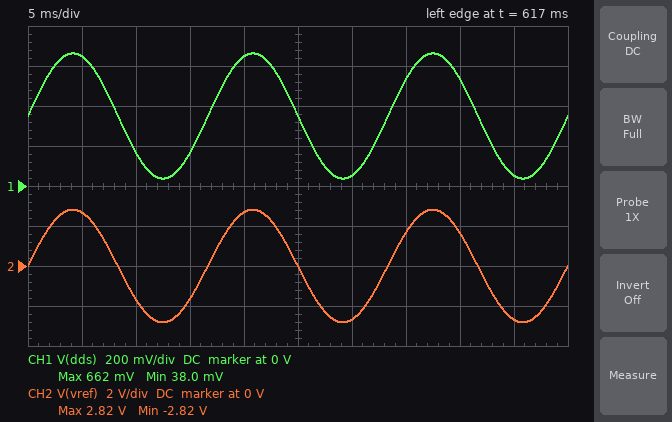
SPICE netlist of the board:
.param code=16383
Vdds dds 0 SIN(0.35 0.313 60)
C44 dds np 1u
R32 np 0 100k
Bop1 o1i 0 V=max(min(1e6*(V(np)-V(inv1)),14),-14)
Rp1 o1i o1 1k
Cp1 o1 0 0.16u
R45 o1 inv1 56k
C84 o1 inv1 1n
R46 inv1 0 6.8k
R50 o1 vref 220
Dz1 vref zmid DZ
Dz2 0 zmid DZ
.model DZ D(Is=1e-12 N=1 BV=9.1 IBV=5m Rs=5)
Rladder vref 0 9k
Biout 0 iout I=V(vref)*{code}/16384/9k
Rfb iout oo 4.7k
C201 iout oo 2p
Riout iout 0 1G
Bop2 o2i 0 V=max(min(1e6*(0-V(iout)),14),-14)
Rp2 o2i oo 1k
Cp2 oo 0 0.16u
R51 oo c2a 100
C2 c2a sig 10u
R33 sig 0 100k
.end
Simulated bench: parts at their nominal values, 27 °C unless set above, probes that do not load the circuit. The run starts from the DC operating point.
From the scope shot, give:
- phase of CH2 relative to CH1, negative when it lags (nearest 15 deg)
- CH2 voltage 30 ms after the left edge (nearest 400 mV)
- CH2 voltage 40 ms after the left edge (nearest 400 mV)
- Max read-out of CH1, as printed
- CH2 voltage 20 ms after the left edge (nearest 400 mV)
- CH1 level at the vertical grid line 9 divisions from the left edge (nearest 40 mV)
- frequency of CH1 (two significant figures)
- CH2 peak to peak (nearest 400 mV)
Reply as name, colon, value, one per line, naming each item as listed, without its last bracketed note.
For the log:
phase of CH2 relative to CH1, negative when it lags: 0 deg
CH2 voltage 30 ms after the left edge: -2.8 V
CH2 voltage 40 ms after the left edge: 1.6 V
Max read-out of CH1, as printed: 662 mV
CH2 voltage 20 ms after the left edge: 2.8 V
CH1 level at the vertical grid line 9 divisions from the left edge: 40 mV
frequency of CH1: 60 Hz
CH2 peak to peak: 5.6 V
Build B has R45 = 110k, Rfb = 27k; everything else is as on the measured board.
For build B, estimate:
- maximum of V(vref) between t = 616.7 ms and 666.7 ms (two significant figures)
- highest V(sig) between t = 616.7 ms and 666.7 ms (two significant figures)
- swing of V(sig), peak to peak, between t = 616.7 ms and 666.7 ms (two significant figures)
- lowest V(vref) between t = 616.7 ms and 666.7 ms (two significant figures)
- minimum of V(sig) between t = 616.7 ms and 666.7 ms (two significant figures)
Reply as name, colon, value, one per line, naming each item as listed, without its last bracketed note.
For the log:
maximum of V(vref) between t = 616.7 ms and 666.7 ms: 5.2 V
highest V(sig) between t = 616.7 ms and 666.7 ms: 13 V
swing of V(sig), peak to peak, between t = 616.7 ms and 666.7 ms: 27 V
lowest V(vref) between t = 616.7 ms and 666.7 ms: -5.2 V
minimum of V(sig) between t = 616.7 ms and 666.7 ms: -13 V
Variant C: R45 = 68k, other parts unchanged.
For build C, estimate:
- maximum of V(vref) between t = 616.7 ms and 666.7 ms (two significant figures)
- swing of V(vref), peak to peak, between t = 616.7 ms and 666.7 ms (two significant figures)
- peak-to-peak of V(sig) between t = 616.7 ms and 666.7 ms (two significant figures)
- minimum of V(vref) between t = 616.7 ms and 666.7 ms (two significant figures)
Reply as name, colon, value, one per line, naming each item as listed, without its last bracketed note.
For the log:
maximum of V(vref) between t = 616.7 ms and 666.7 ms: 3.4 V
swing of V(vref), peak to peak, between t = 616.7 ms and 666.7 ms: 6.7 V
peak-to-peak of V(sig) between t = 616.7 ms and 666.7 ms: 3.5 V
minimum of V(vref) between t = 616.7 ms and 666.7 ms: -3.4 V
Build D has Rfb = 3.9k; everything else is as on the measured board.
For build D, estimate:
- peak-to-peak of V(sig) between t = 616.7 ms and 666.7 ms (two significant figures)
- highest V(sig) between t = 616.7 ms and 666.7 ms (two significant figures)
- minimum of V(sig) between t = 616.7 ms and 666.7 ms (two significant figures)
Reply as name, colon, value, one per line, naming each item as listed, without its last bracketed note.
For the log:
peak-to-peak of V(sig) between t = 616.7 ms and 666.7 ms: 2.4 V
highest V(sig) between t = 616.7 ms and 666.7 ms: 1.2 V
minimum of V(sig) between t = 616.7 ms and 666.7 ms: -1.2 V
